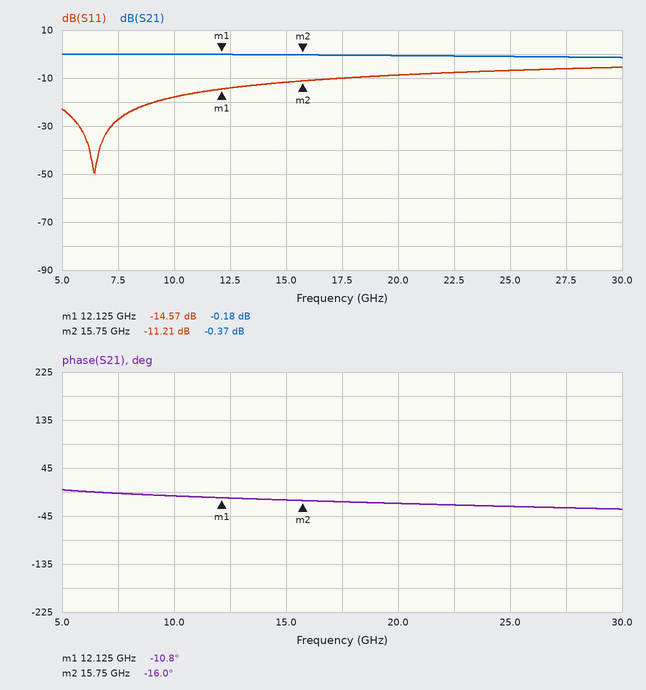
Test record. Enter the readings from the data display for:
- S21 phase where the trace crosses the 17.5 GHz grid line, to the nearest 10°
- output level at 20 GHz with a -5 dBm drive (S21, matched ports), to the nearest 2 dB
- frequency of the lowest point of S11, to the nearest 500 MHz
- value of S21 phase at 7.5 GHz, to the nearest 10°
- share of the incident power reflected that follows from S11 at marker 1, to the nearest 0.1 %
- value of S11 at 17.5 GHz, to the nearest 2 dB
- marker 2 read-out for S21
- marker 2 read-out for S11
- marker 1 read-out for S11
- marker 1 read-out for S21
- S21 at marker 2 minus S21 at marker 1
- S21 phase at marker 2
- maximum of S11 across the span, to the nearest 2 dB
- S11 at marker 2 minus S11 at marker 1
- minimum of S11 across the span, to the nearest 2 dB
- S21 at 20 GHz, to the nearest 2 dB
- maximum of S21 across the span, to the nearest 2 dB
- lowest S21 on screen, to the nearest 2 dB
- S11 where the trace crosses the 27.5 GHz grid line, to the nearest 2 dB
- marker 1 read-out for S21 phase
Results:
-20°
-6 dBm
6.5 GHz
0°
3.5 %
-10 dB
-0.37 dB
-11.21 dB
-14.57 dB
-0.18 dB
-0.19 dB
-16.0°
-6 dB
3.36 dB
-50 dB
0 dB
0 dB
-2 dB
-6 dB
-10.8°
